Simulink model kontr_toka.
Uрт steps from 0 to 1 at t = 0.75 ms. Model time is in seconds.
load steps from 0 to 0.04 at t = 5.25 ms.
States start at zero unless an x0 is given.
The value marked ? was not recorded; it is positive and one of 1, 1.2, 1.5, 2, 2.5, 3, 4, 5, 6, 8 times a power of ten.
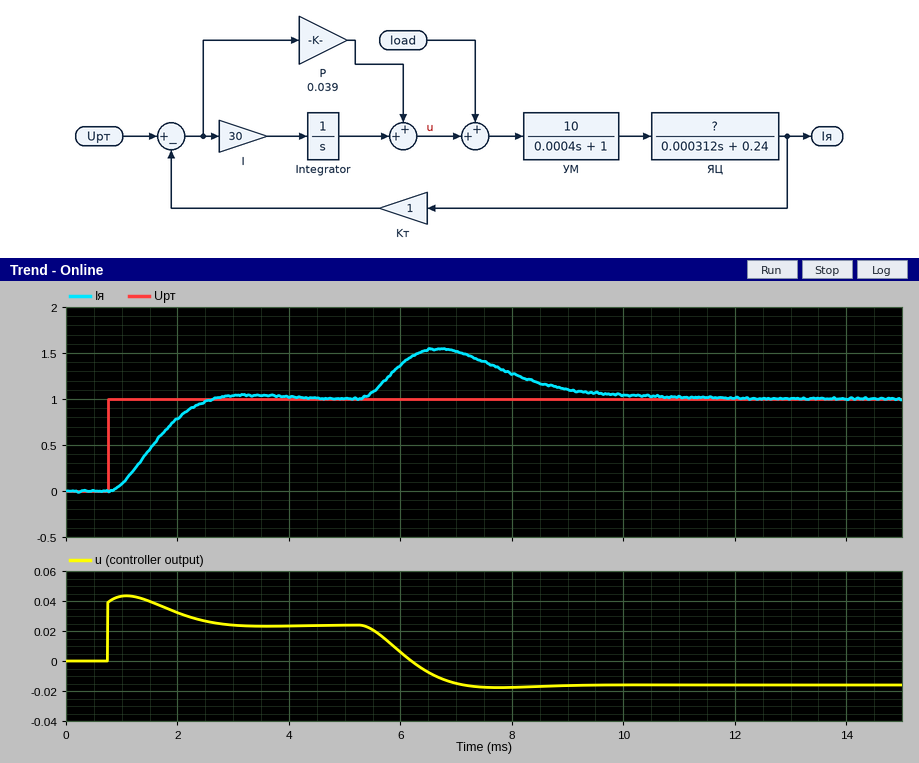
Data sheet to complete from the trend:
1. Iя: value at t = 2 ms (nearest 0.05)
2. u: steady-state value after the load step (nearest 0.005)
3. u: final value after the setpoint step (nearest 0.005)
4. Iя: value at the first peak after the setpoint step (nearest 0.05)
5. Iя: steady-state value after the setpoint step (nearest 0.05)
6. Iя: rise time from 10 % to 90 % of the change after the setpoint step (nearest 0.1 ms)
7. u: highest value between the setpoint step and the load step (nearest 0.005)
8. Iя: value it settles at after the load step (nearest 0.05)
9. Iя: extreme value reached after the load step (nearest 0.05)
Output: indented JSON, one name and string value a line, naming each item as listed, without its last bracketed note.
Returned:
{
  "Iя: value at t = 2 ms": "0.80",
  "u: steady-state value after the load step": "-0.015",
  "u: final value after the setpoint step": "0.025",
  "Iя: value at the first peak after the setpoint step": "1.05",
  "Iя: steady-state value after the setpoint step": "1.00",
  "Iя: rise time from 10 % to 90 % of the change after the setpoint step": "1.2 ms",
  "u: highest value between the setpoint step and the load step": "0.045",
  "Iя: value it settles at after the load step": "1.00",
  "Iя: extreme value reached after the load step": "1.55"
}
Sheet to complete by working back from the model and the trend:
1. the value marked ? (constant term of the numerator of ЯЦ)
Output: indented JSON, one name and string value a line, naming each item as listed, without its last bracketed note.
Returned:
{
  "the value marked ?": "1"
}
